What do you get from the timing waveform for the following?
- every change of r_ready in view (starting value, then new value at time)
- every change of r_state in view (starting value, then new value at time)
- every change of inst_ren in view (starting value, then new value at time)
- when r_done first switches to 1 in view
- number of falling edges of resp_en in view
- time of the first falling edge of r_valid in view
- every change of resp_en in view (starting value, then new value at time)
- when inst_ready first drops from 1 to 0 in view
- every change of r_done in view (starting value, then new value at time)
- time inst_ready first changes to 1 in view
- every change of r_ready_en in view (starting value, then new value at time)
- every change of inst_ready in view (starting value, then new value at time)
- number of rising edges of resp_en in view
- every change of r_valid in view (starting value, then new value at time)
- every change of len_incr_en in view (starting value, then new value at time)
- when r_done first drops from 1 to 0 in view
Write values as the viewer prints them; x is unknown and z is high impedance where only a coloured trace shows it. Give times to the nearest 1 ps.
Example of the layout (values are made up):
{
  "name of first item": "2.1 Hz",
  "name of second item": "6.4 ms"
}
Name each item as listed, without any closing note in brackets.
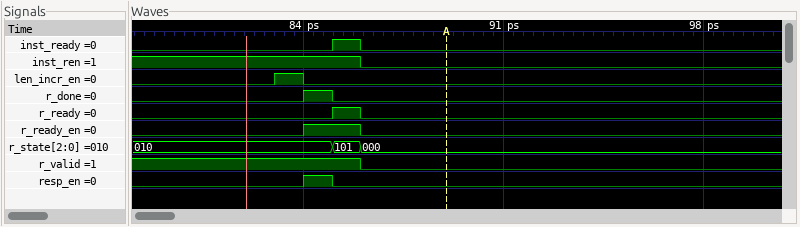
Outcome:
{
  "every change of r_ready in view": "0, 1 at 85 ps, 0 at 86 ps",
  "every change of r_state in view": "010, 101 at 85 ps, 000 at 86 ps",
  "every change of inst_ren in view": "1, 0 at 86 ps",
  "when r_done first switches to 1 in view": "84 ps",
  "number of falling edges of resp_en in view": "1",
  "time of the first falling edge of r_valid in view": "86 ps",
  "every change of resp_en in view": "0, 1 at 84 ps, 0 at 85 ps",
  "when inst_ready first drops from 1 to 0 in view": "86 ps",
  "every change of r_done in view": "0, 1 at 84 ps, 0 at 85 ps",
  "time inst_ready first changes to 1 in view": "85 ps",
  "every change of r_ready_en in view": "0, 1 at 84 ps, 0 at 86 ps",
  "every change of inst_ready in view": "0, 1 at 85 ps, 0 at 86 ps",
  "number of rising edges of resp_en in view": "1",
  "every change of r_valid in view": "1, 0 at 86 ps",
  "every change of len_incr_en in view": "0, 1 at 83 ps, 0 at 84 ps",
  "when r_done first drops from 1 to 0 in view": "85 ps"
}
